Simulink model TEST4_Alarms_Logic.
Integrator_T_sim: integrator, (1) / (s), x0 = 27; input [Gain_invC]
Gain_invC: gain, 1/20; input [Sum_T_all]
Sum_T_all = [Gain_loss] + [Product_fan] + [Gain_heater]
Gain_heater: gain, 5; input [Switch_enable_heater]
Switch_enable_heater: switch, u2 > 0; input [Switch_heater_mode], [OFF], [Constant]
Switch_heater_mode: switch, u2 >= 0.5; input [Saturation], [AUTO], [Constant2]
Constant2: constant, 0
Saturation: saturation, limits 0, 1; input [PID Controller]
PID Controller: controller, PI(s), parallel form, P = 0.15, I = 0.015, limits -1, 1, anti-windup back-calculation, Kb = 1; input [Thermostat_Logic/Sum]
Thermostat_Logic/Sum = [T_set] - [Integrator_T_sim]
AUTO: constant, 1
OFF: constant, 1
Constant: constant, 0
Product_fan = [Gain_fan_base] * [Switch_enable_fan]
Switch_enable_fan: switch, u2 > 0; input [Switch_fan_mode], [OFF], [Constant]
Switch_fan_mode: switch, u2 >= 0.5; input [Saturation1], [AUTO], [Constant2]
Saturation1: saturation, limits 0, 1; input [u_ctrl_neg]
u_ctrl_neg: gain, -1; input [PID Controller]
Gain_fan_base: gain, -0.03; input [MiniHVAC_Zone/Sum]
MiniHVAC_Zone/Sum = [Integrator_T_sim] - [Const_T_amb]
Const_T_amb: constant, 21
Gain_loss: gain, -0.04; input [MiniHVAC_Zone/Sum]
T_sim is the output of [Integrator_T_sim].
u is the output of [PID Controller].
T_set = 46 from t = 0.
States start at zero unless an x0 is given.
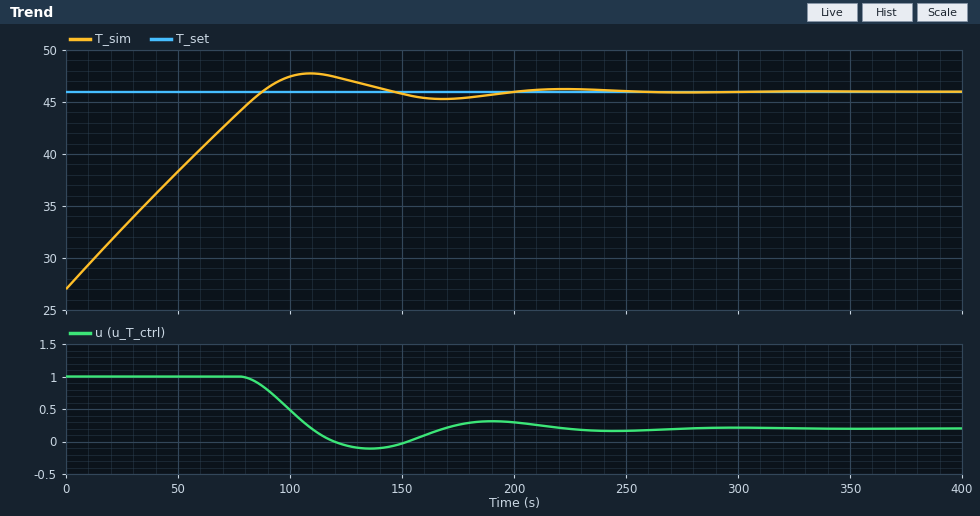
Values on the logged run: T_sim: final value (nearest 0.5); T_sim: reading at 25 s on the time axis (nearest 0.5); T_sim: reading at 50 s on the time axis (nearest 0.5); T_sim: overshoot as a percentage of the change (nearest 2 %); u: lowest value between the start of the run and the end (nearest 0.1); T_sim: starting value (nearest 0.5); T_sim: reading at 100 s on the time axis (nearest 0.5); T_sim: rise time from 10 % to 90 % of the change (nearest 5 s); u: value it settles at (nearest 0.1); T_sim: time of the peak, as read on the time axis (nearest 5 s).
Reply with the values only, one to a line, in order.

46.0
33.0
38.5
10 %
-0.1
27.0
47.5
70 s
0.2
110 s
